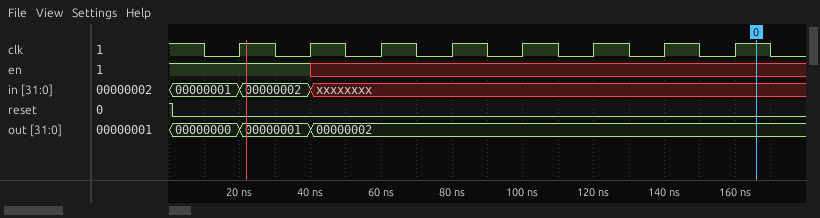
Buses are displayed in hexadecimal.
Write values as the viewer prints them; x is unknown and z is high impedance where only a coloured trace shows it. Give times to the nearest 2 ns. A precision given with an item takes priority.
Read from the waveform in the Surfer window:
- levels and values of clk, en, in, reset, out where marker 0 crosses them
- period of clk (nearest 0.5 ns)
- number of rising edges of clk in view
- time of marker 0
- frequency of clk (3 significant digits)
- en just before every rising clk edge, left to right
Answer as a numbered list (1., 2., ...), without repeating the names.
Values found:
1. clk=1, en=x, in=xxxxxxxx, reset=0, out=00000002
2. 20 ns
3. 8
4. 166 ns
5. 50.0 MHz
6. 1 1 x x x x x x
